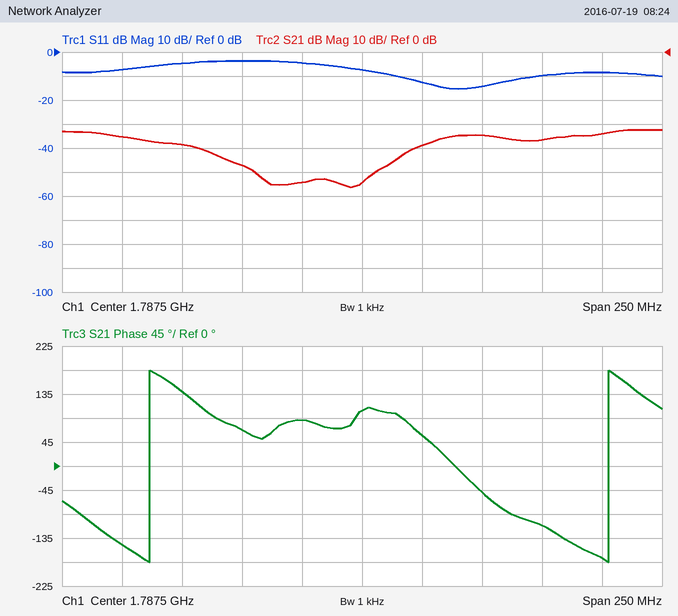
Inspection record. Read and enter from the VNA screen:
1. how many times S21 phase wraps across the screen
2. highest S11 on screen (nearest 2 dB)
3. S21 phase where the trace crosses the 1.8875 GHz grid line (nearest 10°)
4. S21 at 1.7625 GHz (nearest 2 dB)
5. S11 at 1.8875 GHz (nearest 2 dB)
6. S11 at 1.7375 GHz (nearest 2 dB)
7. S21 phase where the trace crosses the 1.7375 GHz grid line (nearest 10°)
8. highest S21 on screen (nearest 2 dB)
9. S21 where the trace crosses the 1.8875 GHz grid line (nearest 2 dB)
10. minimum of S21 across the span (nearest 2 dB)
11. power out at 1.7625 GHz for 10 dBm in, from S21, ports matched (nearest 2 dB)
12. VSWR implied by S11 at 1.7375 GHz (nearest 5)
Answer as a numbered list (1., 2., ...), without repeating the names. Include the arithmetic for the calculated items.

1. 2
2. -4 dB
3. -170°
4. -54 dB
5. -8 dB
6. -4 dB
7. 70°
8. -32 dB
9. -34 dB
10. -56 dB
11. 10 dBm + (-54 dB) = -44 dBm
12. |Γ| = 10^(-4/20) = 0.6310; VSWR = (1 + 0.6310)/(1 − 0.6310) ≈ 4.42, so 5 to the nearest 5
